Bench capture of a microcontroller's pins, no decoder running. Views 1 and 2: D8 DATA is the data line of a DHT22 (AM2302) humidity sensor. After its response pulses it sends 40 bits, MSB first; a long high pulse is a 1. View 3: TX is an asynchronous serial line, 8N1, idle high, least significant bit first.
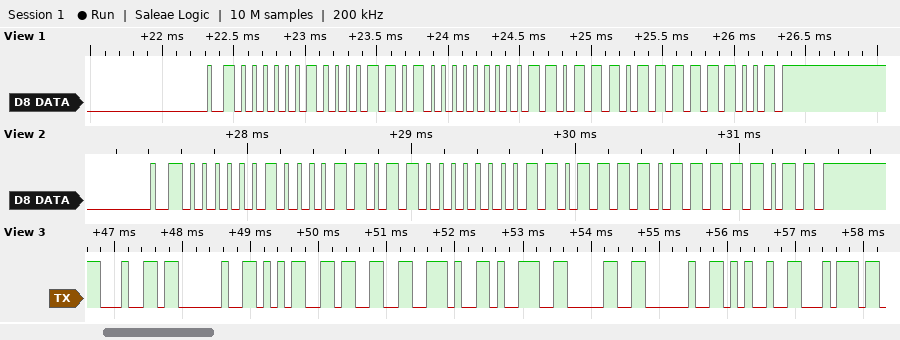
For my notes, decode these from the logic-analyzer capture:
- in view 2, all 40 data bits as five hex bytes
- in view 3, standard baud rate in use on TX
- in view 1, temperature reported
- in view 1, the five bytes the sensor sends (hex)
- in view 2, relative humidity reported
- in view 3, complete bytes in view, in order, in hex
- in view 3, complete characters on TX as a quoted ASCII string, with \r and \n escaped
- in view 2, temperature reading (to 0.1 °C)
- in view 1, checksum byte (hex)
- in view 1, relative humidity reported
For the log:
02 1B 00 DE FB
9600 baud
22.1 °C
02 1A 00 DD F9
53.9 %
0x64 0x20 0x35 0x33 0x2E 0x39 0x30 0x20 0x25 0x74
"d 53.90 %t"
22.2 °C
0xF9
53.8 %
